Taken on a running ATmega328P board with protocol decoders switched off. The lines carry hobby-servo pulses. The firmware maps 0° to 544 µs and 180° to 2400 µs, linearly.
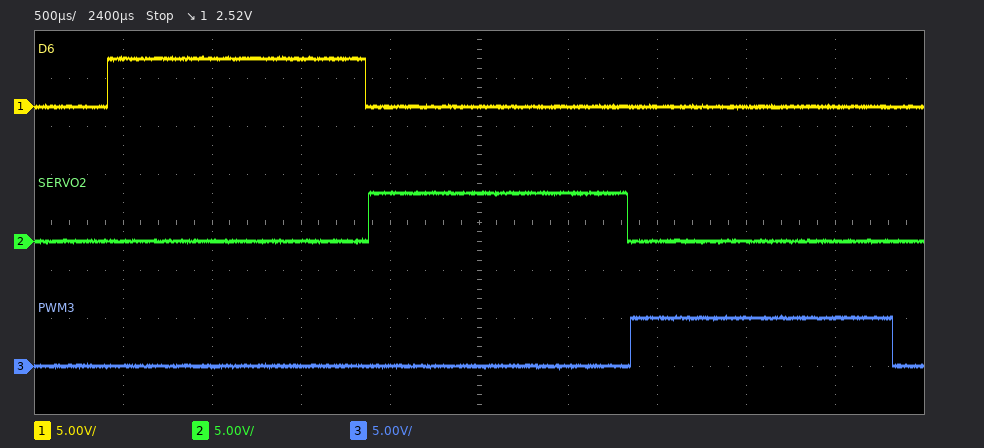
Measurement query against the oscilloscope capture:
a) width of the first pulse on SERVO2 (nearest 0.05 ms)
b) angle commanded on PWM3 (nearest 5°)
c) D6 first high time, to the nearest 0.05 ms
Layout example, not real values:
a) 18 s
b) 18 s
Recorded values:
a) 1.45 ms
b) 90°
c) 1.45 ms
